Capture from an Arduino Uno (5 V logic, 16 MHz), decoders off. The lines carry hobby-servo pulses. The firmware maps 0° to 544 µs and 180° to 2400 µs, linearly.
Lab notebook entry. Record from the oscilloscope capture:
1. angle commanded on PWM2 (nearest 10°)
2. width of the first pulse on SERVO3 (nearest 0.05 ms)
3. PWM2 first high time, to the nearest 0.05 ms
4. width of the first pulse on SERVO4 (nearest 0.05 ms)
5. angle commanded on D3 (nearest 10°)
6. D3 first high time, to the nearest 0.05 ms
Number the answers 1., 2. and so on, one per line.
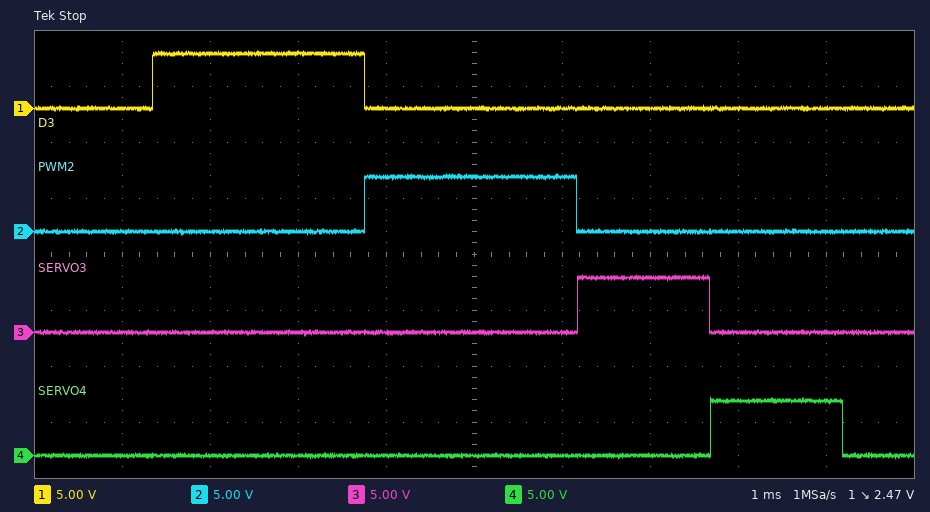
1. 180°
2. 1.50 ms
3. 2.40 ms
4. 1.50 ms
5. 180°
6. 2.40 ms
